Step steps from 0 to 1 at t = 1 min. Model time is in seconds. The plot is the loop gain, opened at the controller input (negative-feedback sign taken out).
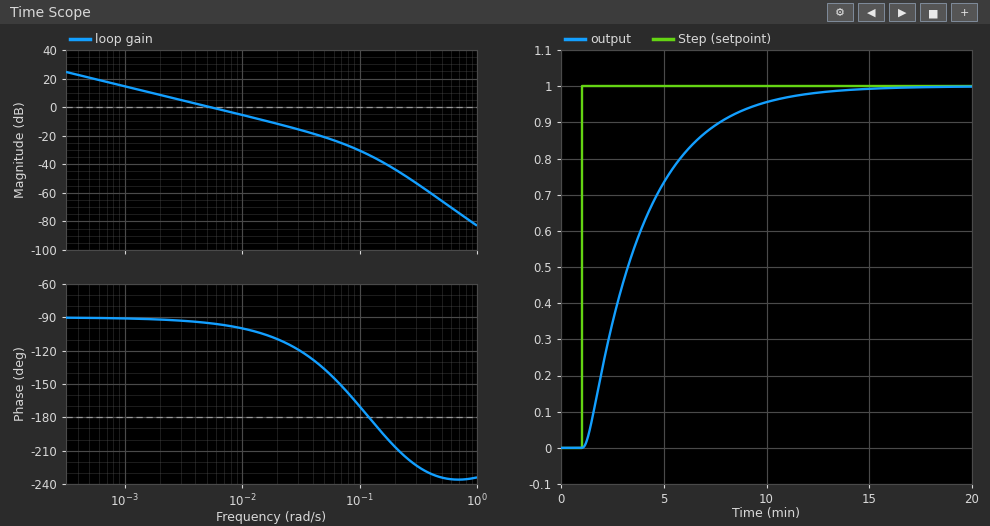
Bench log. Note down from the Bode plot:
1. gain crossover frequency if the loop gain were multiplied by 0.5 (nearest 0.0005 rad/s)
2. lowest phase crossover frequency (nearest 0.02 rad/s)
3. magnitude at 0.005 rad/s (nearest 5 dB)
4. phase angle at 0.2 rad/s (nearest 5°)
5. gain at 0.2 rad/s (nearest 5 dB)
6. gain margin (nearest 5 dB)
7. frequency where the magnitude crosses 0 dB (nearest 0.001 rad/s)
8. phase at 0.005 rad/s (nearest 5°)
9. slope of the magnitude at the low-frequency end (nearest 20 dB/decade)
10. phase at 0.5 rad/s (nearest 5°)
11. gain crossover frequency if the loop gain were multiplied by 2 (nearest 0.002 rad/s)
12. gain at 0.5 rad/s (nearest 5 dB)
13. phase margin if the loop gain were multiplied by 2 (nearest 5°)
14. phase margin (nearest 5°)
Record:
0.0025 rad/s
0.12 rad/s
0 dB
-205°
-45 dB
35 dB
0.005 rad/s
-95°
-20 dB/decade
-235°
0.010 rad/s
-65 dB
80°
85°
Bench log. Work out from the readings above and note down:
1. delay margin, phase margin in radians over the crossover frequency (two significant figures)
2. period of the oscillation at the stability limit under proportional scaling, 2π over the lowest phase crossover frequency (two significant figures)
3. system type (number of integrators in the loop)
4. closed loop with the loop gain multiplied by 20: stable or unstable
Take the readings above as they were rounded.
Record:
300 s
52 s
1
stable
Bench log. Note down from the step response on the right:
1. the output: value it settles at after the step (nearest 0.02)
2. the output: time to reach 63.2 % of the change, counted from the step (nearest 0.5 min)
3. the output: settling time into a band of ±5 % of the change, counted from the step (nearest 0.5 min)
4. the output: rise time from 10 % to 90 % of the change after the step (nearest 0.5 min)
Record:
1.00
3.0 min
8.5 min
6.0 min
